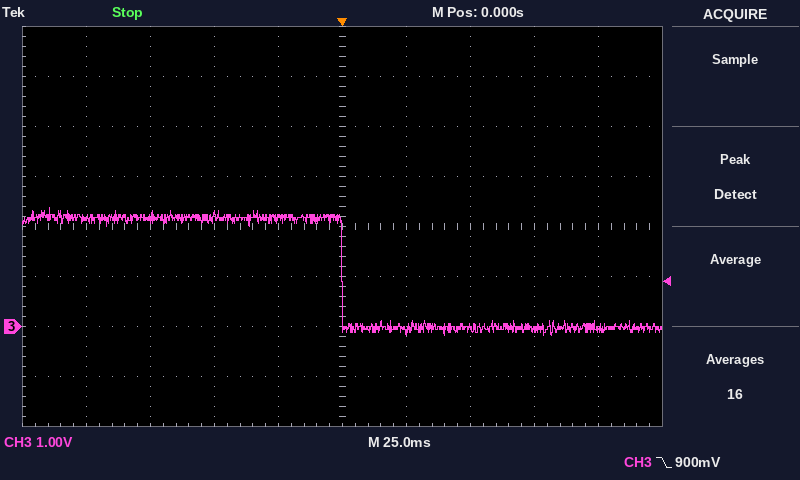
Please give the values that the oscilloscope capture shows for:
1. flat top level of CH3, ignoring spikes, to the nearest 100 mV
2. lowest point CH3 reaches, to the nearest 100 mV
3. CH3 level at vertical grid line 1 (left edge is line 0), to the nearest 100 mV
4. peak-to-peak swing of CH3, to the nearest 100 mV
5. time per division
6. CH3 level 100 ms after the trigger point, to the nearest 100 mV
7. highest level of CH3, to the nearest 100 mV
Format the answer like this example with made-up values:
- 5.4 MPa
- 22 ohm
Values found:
- 2.2 V
- -200 mV
- 2.2 V
- 2.6 V
- 25 ms
- 0.0 V
- 2.4 V
